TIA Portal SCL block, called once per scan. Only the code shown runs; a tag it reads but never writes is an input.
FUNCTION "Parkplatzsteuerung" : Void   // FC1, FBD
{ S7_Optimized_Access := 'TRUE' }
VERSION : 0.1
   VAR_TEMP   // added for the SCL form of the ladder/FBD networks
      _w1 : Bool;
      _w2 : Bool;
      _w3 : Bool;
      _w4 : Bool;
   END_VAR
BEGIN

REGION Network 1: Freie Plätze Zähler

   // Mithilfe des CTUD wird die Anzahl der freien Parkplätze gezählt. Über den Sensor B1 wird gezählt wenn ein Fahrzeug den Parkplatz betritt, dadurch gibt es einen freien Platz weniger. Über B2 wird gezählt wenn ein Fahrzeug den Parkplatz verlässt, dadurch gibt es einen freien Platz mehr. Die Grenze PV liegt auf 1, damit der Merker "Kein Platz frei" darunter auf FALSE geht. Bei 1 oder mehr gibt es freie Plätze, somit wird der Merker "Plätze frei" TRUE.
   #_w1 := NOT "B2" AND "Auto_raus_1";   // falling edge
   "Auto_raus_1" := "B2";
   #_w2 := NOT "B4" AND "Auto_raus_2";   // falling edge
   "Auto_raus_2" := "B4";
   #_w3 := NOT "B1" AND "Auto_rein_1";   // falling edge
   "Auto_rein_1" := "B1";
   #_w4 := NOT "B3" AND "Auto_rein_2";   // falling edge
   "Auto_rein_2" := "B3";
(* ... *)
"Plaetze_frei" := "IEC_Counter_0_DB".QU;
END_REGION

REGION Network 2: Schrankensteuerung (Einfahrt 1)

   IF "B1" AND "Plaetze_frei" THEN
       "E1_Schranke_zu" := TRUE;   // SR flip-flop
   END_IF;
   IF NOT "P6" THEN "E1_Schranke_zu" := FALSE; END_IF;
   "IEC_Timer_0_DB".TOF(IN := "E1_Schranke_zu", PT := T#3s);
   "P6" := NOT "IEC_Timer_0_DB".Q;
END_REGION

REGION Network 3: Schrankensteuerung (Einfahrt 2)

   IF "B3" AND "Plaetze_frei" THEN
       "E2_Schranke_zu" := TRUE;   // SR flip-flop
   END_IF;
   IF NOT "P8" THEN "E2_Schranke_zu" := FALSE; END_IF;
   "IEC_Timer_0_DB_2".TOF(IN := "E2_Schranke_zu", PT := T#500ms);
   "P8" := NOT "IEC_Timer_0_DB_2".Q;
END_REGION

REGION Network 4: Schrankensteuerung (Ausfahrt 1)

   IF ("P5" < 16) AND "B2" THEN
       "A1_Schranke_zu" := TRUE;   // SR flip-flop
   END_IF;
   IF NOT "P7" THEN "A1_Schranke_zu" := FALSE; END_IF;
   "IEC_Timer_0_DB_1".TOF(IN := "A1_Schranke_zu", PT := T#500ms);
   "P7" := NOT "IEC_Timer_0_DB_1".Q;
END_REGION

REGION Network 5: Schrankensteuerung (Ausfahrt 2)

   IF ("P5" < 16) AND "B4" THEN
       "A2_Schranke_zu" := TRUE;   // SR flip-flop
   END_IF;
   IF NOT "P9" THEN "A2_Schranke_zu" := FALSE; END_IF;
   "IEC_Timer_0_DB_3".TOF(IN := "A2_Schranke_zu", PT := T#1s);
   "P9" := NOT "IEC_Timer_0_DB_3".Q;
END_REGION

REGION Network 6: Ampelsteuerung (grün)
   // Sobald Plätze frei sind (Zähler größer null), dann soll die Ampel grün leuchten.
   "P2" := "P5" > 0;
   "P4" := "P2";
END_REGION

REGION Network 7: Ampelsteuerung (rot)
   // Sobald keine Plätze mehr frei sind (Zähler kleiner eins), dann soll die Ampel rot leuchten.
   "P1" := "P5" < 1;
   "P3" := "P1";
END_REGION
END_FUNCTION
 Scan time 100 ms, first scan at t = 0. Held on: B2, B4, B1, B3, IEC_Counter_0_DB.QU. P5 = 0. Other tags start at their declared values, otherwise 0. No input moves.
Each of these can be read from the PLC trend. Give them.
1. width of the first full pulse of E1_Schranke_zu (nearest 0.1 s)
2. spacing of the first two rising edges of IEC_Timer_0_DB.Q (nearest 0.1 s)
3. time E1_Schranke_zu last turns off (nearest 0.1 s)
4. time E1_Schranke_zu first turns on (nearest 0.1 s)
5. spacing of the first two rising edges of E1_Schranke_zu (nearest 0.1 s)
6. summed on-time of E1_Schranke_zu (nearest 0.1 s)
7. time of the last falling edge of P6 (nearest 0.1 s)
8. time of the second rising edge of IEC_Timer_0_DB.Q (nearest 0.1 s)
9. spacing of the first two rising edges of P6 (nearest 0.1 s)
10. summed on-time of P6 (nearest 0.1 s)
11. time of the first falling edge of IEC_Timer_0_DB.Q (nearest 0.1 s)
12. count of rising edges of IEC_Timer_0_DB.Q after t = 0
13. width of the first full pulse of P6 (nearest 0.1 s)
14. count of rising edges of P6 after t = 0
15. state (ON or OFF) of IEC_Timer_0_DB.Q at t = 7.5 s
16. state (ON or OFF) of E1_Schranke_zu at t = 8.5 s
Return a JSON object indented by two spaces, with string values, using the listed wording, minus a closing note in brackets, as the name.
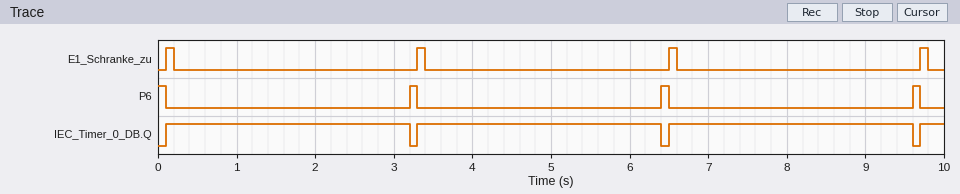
{
  "width of the first full pulse of E1_Schranke_zu": "0.1 s",
  "spacing of the first two rising edges of IEC_Timer_0_DB.Q": "3.2 s",
  "time E1_Schranke_zu last turns off": "9.8 s",
  "time E1_Schranke_zu first turns on": "0.1 s",
  "spacing of the first two rising edges of E1_Schranke_zu": "3.2 s",
  "summed on-time of E1_Schranke_zu": "0.4 s",
  "time of the last falling edge of P6": "9.7 s",
  "time of the second rising edge of IEC_Timer_0_DB.Q": "3.3 s",
  "spacing of the first two rising edges of P6": "3.2 s",
  "summed on-time of P6": "0.4 s",
  "time of the first falling edge of IEC_Timer_0_DB.Q": "3.2 s",
  "count of rising edges of IEC_Timer_0_DB.Q after t = 0": "4",
  "width of the first full pulse of P6": "0.1 s",
  "count of rising edges of P6 after t = 0": "3",
  "state (ON or OFF) of IEC_Timer_0_DB.Q at t = 7.5 s": "ON",
  "state (ON or OFF) of E1_Schranke_zu at t = 8.5 s": "OFF"
}
